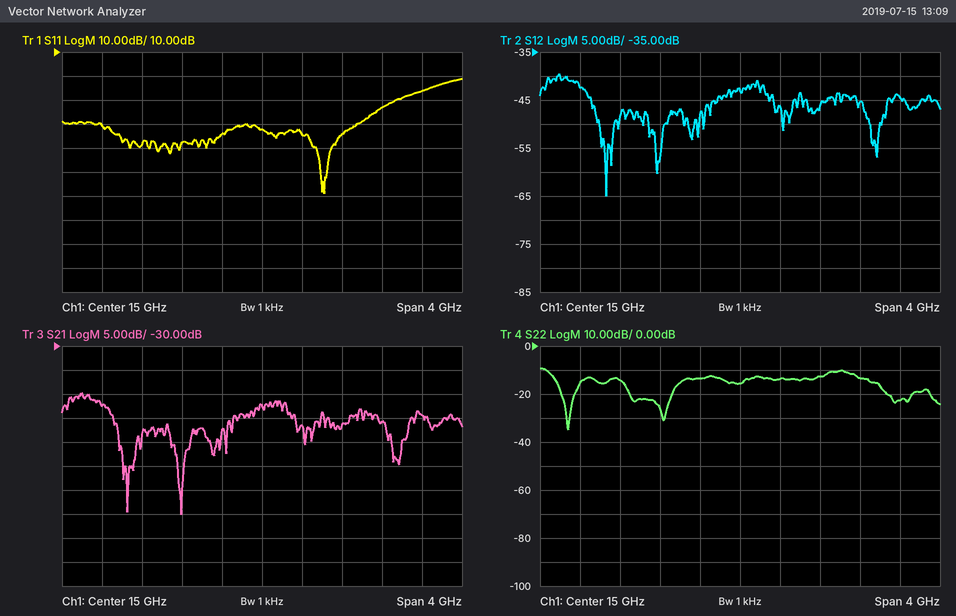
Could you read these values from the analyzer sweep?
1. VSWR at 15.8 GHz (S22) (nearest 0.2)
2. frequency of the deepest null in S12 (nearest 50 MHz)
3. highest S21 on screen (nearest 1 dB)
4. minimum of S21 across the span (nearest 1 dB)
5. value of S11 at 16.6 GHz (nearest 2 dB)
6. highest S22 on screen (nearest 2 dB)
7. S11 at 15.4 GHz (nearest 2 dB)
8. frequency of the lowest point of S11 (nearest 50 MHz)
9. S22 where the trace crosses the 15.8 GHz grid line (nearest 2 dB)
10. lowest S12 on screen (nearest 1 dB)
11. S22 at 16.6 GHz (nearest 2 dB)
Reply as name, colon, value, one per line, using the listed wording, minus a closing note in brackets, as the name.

VSWR at 15.8 GHz (S22): 1.6
frequency of the deepest null in S12: 13.65 GHz
highest S21 on screen: -40 dB
minimum of S21 across the span: -65 dB
value of S11 at 16.6 GHz: -6 dB
highest S22 on screen: -10 dB
S11 at 15.4 GHz: -24 dB
frequency of the lowest point of S11: 15.60 GHz
S22 where the trace crosses the 15.8 GHz grid line: -12 dB
lowest S12 on screen: -65 dB
S22 at 16.6 GHz: -22 dB
